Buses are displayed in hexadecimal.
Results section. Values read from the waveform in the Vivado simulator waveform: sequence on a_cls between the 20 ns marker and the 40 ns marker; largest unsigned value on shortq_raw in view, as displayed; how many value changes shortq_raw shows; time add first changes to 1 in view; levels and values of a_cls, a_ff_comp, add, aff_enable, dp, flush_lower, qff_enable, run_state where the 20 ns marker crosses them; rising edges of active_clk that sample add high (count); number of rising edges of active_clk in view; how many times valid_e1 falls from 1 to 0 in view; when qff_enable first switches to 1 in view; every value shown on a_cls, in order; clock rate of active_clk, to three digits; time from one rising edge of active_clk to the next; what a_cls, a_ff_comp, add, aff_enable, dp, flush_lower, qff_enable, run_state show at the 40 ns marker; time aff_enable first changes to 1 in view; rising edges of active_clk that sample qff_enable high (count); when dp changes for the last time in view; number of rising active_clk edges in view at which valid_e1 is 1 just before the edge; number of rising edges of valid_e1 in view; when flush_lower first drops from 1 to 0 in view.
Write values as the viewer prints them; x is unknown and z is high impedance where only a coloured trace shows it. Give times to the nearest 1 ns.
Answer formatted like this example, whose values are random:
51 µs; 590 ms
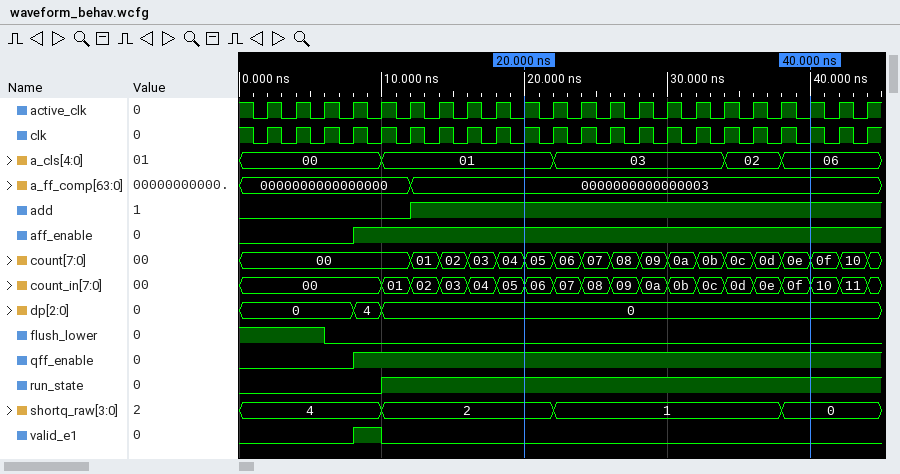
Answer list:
01, 03, 02, 06; 4; 3; 12 ns; a_cls=01, a_ff_comp=0000000000000003, add=1, aff_enable=1, dp=0, flush_lower=0, qff_enable=1, run_state=1; 16; 22; 1; 8 ns; 00, 01, 03, 02, 06; 500 MHz; 2 ns; a_cls=06, a_ff_comp=0000000000000003, add=1, aff_enable=1, dp=0, flush_lower=0, qff_enable=1, run_state=1; 8 ns; 18; 10 ns; 1; 1; 6 ns
